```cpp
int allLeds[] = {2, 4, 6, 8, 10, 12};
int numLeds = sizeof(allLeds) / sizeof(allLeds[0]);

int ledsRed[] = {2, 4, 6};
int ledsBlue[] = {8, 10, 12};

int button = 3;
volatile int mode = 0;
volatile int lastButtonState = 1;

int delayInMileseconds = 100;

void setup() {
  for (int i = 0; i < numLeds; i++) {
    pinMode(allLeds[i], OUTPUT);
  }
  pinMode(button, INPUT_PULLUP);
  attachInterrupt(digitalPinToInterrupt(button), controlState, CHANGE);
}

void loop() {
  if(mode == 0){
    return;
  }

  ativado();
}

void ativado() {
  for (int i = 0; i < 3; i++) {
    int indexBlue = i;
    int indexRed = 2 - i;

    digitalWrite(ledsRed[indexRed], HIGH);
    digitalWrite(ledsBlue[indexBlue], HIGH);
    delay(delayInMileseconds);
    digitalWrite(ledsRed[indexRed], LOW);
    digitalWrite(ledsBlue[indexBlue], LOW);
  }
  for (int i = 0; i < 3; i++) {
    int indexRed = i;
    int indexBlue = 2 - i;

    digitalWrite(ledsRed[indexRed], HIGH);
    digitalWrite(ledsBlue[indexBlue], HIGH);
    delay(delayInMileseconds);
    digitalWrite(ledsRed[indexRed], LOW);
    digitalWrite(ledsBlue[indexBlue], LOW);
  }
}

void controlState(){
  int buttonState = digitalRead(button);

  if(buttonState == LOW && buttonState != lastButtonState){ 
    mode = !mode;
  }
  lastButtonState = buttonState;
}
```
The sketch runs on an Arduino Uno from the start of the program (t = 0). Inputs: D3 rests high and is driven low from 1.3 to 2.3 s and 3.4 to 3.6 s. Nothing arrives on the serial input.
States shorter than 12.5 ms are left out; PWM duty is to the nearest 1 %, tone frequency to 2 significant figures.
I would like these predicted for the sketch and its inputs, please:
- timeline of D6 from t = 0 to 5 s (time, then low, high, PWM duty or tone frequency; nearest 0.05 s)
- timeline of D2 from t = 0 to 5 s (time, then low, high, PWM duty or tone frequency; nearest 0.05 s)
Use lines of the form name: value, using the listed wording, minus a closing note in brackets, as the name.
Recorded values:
timeline of D6 from t = 0 to 5 s: 0 s low; 1.3 s high; 1.4 s low; 1.8 s high; 2 s low; 2.4 s high; 2.6 s low; 3 s high; 3.2 s low; 3.6 s high; 3.7 s low
timeline of D2 from t = 0 to 5 s: 0 s low; 1.5 s high; 1.7 s low; 2.1 s high; 2.3 s low; 2.7 s high; 2.9 s low; 3.3 s high; 3.5 s low
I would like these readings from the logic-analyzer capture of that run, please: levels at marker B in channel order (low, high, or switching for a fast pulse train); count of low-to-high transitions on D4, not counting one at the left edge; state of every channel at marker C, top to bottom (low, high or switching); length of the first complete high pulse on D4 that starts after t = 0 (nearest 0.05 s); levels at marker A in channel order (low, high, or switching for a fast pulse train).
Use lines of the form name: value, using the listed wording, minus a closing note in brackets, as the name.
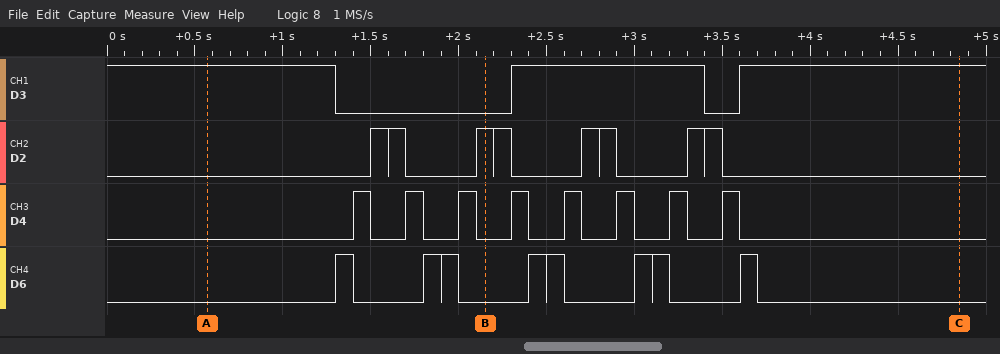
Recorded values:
levels at marker B in channel order: D3 low, D2 high, D4 low, D6 low
count of low-to-high transitions on D4, not counting one at the left edge: 8
state of every channel at marker C, top to bottom: D3 high, D2 low, D4 low, D6 low
length of the first complete high pulse on D4 that starts after t = 0: 0.10 s
levels at marker A in channel order: D3 high, D2 low, D4 low, D6 low
